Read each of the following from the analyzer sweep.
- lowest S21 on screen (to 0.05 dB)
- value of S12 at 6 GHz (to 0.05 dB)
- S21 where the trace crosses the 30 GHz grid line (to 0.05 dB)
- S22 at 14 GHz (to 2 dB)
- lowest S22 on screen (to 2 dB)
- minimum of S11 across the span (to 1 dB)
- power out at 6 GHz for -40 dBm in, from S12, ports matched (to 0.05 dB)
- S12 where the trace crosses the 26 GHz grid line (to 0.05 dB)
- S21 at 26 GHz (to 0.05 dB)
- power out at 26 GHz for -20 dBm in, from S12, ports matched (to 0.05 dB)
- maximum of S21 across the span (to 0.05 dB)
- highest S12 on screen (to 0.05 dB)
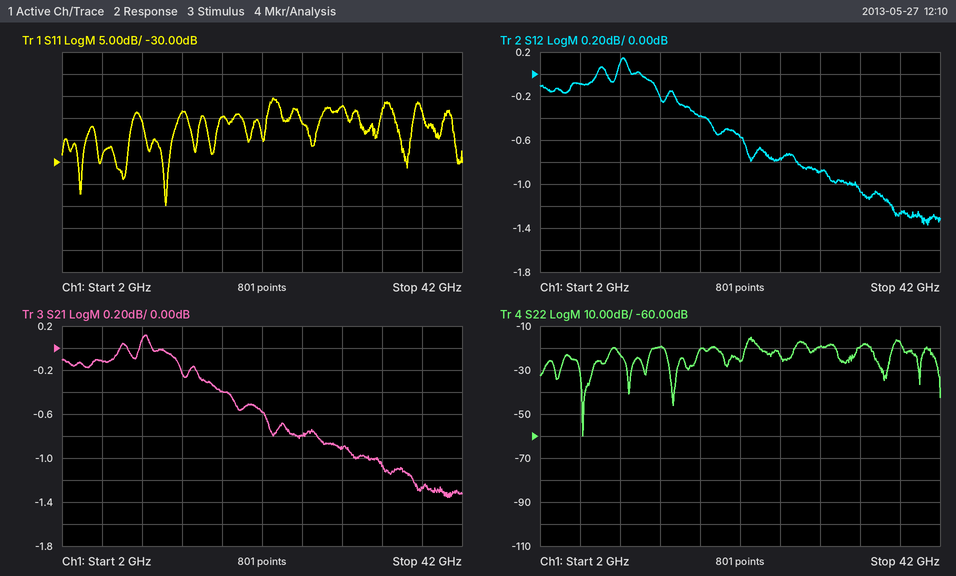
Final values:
-1.35 dB
-0.10 dB
-0.90 dB
-20 dB
-60 dB
-40 dB
-40.10 dBm
-0.75 dB
-0.80 dB
-20.75 dBm
0.10 dB
0.15 dB
